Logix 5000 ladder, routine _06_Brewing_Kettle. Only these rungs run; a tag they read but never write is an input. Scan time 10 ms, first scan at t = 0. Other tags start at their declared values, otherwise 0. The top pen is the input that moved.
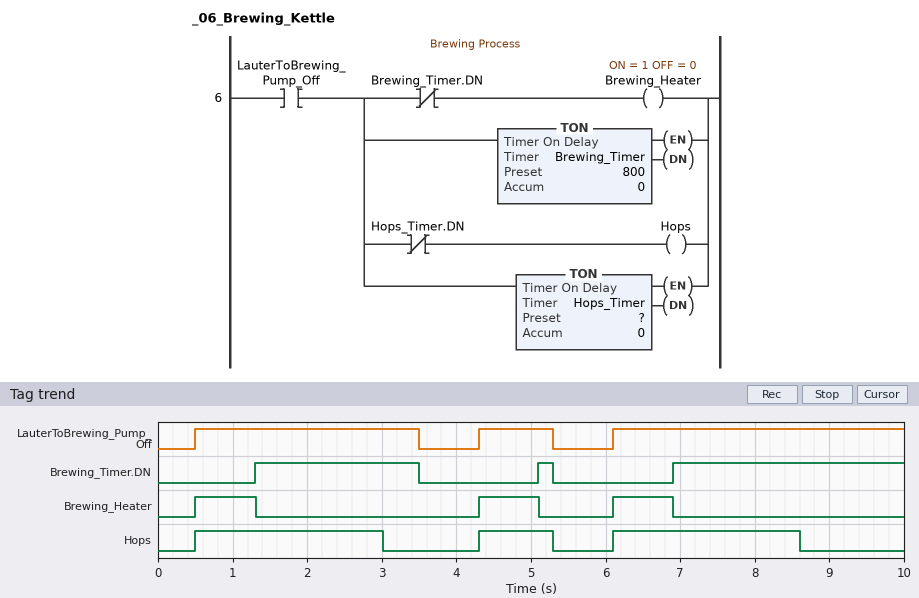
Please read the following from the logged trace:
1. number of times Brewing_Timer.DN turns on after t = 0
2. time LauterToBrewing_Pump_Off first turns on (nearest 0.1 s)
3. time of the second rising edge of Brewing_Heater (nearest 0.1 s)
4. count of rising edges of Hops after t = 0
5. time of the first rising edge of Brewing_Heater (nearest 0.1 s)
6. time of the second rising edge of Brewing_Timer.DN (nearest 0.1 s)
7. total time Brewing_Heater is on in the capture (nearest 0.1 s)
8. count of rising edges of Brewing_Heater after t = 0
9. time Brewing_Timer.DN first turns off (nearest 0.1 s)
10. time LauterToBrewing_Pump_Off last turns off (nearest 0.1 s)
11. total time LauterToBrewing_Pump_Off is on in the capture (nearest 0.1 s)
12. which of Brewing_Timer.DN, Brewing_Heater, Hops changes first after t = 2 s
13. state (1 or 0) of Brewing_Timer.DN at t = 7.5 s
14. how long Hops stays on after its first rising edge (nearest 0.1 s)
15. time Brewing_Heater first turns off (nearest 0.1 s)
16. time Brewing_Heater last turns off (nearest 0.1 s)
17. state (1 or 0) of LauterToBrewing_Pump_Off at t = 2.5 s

3
0.5 s
4.3 s
3
0.5 s
5.1 s
2.4 s
3
3.5 s
5.3 s
7.9 s
Hops
1
2.5 s
1.3 s
6.9 s
1
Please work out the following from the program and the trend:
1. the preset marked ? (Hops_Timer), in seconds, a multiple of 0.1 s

2.5 s
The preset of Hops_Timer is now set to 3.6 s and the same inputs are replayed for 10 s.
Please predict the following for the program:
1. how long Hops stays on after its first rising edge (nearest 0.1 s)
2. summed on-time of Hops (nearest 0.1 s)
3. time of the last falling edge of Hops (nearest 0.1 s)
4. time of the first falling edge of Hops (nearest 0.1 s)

3.0 s
7.6 s
9.7 s
3.5 s
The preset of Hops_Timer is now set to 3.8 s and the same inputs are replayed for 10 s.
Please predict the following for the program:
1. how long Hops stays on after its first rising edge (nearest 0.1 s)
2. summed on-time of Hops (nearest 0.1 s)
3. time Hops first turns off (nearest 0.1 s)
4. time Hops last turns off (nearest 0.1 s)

3.0 s
7.8 s
3.5 s
9.9 s
